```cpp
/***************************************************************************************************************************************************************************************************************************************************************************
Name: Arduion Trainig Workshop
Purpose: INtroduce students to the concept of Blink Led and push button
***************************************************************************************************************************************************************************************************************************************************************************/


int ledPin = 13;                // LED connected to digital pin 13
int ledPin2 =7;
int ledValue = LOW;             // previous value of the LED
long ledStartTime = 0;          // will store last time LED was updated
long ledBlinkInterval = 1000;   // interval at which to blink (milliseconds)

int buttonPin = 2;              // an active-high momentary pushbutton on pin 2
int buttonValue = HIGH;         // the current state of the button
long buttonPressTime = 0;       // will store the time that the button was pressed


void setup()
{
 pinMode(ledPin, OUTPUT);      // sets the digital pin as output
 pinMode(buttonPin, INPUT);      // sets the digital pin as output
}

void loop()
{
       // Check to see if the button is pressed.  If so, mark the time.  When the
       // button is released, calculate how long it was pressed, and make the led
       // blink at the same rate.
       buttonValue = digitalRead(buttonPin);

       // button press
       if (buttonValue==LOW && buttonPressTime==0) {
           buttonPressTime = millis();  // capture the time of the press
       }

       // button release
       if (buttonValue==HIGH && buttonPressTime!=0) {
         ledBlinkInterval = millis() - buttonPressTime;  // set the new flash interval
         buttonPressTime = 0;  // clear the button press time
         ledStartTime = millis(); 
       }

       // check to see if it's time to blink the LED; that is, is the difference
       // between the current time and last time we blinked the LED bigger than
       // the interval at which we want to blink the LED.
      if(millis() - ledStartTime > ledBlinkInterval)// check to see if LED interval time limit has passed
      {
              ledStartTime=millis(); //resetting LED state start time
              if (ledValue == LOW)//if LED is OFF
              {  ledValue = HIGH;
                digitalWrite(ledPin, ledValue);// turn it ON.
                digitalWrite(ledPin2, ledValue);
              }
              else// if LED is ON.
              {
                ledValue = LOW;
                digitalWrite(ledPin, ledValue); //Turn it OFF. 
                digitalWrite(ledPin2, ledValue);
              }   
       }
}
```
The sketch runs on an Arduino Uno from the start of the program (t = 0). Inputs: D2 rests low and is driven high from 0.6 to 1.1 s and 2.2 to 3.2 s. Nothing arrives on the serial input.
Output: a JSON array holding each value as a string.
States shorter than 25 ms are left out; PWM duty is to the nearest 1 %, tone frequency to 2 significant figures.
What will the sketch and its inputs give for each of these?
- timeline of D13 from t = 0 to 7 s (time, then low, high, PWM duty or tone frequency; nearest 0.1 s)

["0 s low; 1.2 s high; 1.8 s low; 3.3 s high; 4.4 s low; 5.5 s high; 6.6 s low"]
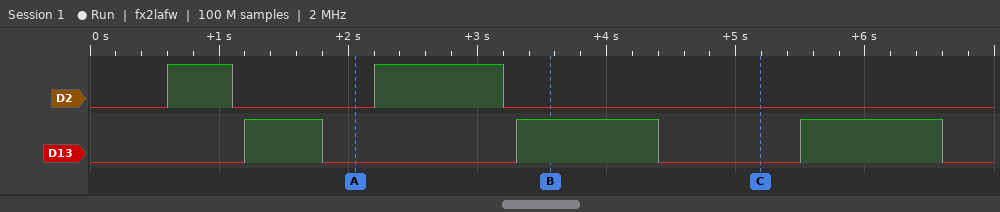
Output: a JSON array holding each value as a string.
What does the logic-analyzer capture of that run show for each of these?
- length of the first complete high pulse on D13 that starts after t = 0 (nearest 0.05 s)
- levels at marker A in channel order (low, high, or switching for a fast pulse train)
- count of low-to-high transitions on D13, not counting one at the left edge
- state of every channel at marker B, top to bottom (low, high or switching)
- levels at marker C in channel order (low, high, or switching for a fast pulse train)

["0.60 s", "D2 low, D13 low", "3", "D2 low, D13 high", "D2 low, D13 low"]
